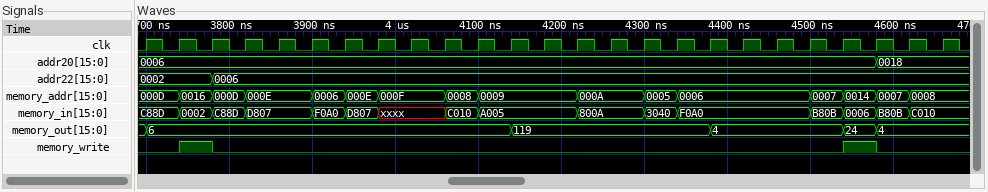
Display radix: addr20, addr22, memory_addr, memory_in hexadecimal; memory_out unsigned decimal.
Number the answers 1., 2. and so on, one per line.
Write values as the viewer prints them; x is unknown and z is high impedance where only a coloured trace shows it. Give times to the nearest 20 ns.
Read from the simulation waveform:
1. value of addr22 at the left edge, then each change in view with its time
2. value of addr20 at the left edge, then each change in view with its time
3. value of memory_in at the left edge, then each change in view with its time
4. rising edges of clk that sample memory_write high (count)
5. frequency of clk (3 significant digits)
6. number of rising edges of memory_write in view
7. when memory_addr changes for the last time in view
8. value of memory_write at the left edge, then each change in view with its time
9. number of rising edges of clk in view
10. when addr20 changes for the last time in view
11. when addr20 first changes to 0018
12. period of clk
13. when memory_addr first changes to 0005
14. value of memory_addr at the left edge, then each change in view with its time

1. 0002, 0006 at 3780 ns
2. 0006, 0018 at 4580 ns
3. C88D, 0002 at 3740 ns, C88D at 3780 ns, D807 at 3820 ns, F0A0 at 3900 ns, D807 at 3940 ns, xxxx at 3980 ns, C010 at 4060 ns, A005 at 4100 ns, 800A at 4220 ns, 3040 at 4300 ns, F0A0 at 4340 ns, B80B at 4500 ns, 0006 at 4540 ns, B80B at 4580 ns, C010 at 4620 ns
4. 2
5. 25.0 MHz
6. 2
7. 4620 ns
8. 0, 1 at 3740 ns, 0 at 3780 ns, 1 at 4540 ns, 0 at 4580 ns
9. 25
10. 4580 ns
11. 4580 ns
12. 40 ns
13. 4300 ns
14. 000D, 0016 at 3740 ns, 000D at 3780 ns, 000E at 3820 ns, 0006 at 3900 ns, 000E at 3940 ns, 000F at 3980 ns, 0008 at 4060 ns, 0009 at 4100 ns, 000A at 4220 ns, 0005 at 4300 ns, 0006 at 4340 ns, 0007 at 4500 ns, 0014 at 4540 ns, 0007 at 4580 ns, 0008 at 4620 ns
